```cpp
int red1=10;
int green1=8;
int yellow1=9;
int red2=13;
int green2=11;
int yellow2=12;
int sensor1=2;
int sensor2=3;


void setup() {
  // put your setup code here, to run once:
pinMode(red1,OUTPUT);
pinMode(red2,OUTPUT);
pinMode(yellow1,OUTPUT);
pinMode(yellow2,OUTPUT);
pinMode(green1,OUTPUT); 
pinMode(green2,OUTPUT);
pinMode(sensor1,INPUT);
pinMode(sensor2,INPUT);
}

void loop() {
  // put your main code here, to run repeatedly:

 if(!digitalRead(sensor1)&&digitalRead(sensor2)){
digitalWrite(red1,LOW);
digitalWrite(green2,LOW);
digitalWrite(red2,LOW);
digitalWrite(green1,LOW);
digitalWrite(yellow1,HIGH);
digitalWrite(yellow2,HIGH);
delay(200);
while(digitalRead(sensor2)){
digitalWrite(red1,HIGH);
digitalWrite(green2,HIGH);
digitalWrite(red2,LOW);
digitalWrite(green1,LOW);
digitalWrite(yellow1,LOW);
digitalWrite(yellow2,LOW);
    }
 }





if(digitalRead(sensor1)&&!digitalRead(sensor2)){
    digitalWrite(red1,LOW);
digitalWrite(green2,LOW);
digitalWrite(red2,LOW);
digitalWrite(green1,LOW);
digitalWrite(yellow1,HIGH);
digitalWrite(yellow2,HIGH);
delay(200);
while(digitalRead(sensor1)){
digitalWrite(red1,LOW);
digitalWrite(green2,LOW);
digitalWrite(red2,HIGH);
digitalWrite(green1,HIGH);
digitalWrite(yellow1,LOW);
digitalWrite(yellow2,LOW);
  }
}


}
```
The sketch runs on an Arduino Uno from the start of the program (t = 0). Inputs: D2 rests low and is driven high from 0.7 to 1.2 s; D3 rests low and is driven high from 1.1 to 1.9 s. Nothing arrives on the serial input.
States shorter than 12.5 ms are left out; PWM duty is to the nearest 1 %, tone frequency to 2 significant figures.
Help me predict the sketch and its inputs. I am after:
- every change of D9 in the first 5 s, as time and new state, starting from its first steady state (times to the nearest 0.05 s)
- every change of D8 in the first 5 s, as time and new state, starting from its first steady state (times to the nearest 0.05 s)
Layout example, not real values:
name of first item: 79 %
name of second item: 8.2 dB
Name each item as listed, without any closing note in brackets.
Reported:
every change of D9 in the first 5 s, as time and new state, starting from its first steady state: 0 s low; 0.7 s high; 0.9 s low; 1.2 s high; 1.4 s low
every change of D8 in the first 5 s, as time and new state, starting from its first steady state: 0 s low; 0.9 s high; 1.2 s low
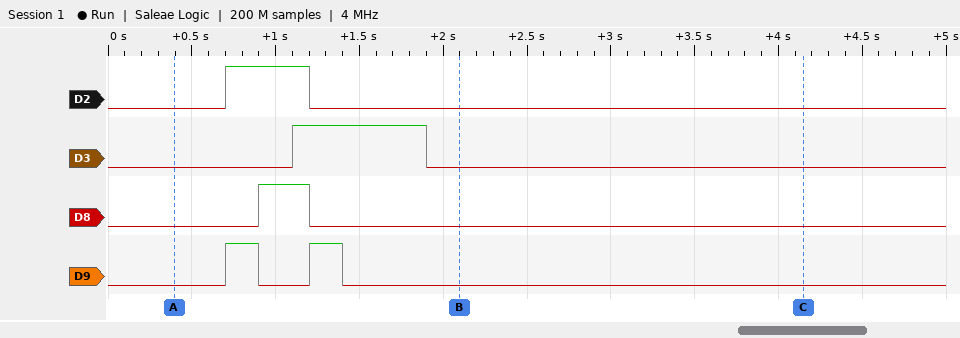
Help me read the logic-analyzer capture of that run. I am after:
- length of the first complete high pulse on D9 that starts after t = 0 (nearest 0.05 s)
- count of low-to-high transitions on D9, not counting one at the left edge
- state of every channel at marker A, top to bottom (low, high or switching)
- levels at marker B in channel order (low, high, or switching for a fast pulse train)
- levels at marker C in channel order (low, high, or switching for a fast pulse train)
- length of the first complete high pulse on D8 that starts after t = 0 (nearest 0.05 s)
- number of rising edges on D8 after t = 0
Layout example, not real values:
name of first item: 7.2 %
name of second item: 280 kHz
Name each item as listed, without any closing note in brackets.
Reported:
length of the first complete high pulse on D9 that starts after t = 0: 0.20 s
count of low-to-high transitions on D9, not counting one at the left edge: 2
state of every channel at marker A, top to bottom: D2 low, D3 low, D8 low, D9 low
levels at marker B in channel order: D2 low, D3 low, D8 low, D9 low
levels at marker C in channel order: D2 low, D3 low, D8 low, D9 low
length of the first complete high pulse on D8 that starts after t = 0: 0.30 s
number of rising edges on D8 after t = 0: 1
